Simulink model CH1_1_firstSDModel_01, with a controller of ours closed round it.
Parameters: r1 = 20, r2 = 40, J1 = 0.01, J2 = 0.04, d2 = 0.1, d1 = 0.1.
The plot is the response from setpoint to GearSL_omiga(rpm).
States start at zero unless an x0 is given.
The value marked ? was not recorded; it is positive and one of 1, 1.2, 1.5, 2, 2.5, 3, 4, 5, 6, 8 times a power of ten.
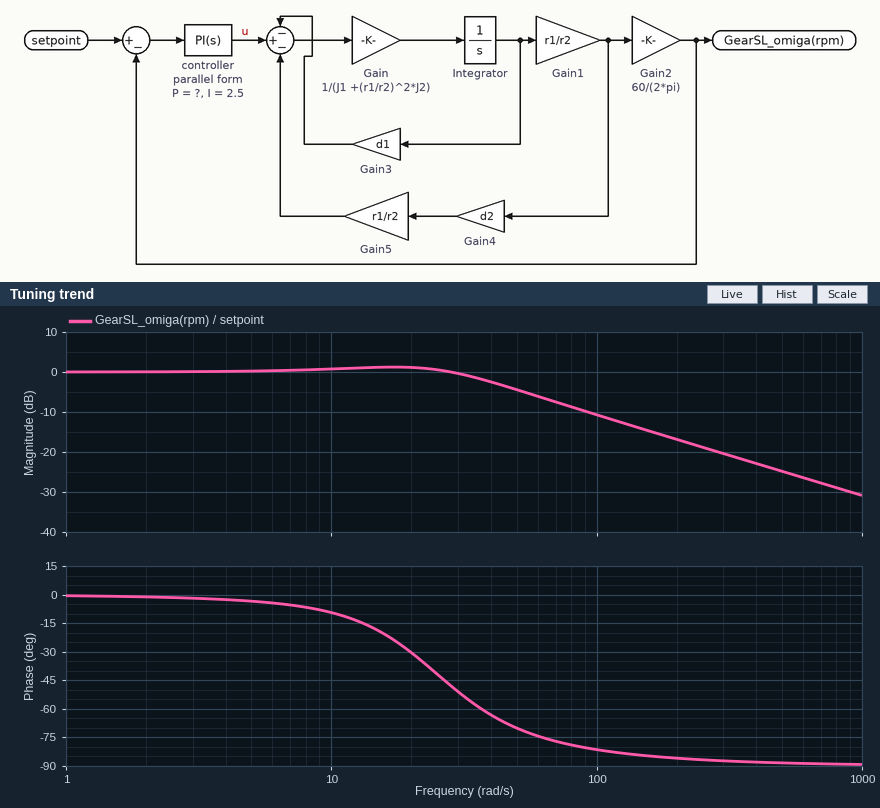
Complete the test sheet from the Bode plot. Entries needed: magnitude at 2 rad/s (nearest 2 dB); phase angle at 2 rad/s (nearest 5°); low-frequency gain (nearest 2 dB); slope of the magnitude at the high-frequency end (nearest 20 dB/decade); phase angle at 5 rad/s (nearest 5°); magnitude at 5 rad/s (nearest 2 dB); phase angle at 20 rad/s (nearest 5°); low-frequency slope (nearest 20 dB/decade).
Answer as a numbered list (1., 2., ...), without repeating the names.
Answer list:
1. 0 dB
2. 0°
3. 0 dB
4. -20 dB/decade
5. -5°
6. 0 dB
7. -30°
8. 0 dB/decade
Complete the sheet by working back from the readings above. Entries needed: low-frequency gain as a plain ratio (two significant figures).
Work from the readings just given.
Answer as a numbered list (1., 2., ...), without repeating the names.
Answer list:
1. 1.0
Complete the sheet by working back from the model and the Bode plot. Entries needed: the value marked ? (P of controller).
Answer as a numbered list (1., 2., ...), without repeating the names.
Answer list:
1. 0.12
